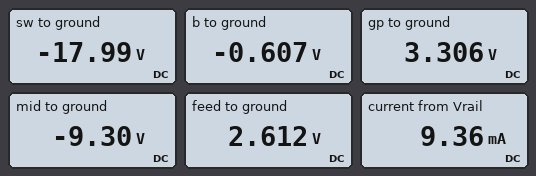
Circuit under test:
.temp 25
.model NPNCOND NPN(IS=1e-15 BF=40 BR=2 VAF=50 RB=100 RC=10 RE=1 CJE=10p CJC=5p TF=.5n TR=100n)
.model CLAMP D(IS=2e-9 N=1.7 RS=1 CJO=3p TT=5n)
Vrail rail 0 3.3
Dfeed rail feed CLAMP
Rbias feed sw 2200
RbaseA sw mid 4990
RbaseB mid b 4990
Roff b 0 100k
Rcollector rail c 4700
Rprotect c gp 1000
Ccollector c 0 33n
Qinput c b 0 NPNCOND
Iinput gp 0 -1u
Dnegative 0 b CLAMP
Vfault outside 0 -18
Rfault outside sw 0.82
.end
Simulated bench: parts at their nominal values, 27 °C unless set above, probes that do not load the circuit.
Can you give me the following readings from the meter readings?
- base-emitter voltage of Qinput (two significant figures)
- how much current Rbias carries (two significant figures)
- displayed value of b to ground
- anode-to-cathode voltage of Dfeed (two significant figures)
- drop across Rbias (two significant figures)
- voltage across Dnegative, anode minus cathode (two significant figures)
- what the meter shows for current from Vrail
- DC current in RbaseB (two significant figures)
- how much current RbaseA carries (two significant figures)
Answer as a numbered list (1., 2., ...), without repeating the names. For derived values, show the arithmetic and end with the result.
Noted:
1. -607 mV = -610 mV
2. (2.612 V - (-17.99 V)) / 2.2 kΩ = 9.4 mA
3. -0.607 V
4. 3.3 V - 2.612 V = 690 mV
5. 2.612 V - (-17.99 V) = 21 V
6. 0 V - (-607 mV) = 610 mV
7. 9.36 mA
8. (-607 mV - (-9.3 V)) / 4.99 kΩ = 1.7 mA
9. (-9.3 V - (-17.99 V)) / 4.99 kΩ = 1.7 mA
